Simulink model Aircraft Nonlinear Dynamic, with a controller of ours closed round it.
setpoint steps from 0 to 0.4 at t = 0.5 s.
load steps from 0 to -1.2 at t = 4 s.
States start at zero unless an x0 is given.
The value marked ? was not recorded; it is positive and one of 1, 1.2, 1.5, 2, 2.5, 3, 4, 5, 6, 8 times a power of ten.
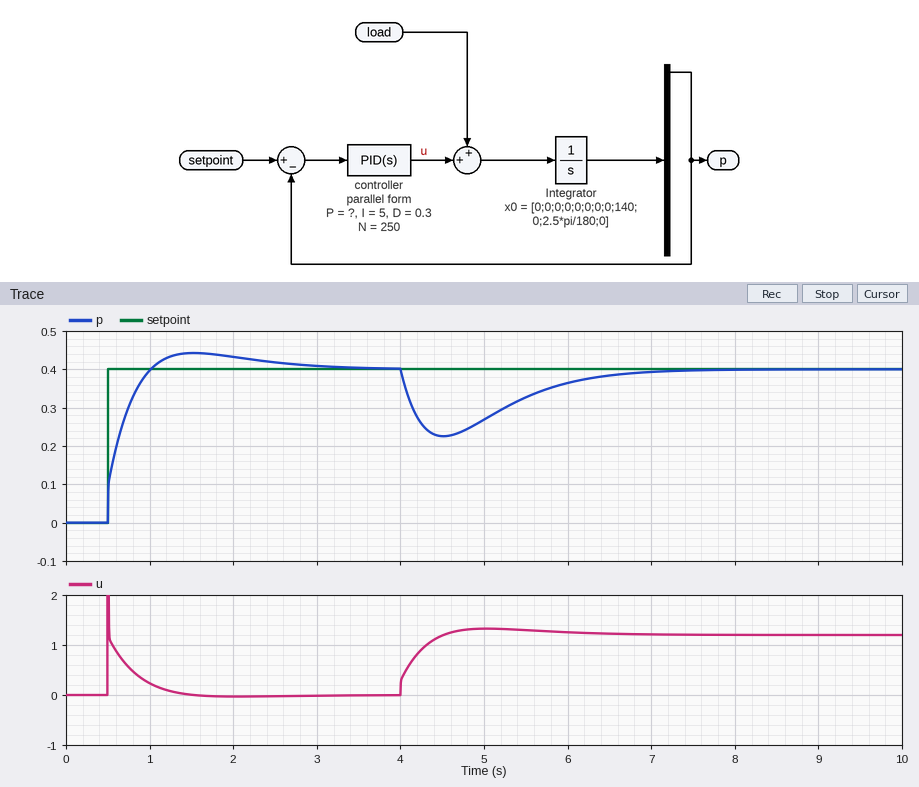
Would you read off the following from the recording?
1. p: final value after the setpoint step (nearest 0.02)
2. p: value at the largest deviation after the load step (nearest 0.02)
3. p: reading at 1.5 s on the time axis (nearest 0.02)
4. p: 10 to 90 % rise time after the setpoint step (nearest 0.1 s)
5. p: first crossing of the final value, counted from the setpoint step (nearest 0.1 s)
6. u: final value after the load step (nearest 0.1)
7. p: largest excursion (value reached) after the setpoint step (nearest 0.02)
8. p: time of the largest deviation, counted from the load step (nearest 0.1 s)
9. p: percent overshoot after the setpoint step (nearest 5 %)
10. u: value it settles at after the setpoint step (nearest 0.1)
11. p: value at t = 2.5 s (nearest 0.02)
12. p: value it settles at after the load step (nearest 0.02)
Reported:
0.40
0.22
0.44
0.4 s
0.5 s
1.2
0.44
0.5 s
10 %
0.0
0.42
0.40
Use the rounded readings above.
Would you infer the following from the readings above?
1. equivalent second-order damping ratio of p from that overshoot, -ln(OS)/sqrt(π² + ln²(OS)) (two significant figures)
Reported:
0.59
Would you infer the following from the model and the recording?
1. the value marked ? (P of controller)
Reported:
5
